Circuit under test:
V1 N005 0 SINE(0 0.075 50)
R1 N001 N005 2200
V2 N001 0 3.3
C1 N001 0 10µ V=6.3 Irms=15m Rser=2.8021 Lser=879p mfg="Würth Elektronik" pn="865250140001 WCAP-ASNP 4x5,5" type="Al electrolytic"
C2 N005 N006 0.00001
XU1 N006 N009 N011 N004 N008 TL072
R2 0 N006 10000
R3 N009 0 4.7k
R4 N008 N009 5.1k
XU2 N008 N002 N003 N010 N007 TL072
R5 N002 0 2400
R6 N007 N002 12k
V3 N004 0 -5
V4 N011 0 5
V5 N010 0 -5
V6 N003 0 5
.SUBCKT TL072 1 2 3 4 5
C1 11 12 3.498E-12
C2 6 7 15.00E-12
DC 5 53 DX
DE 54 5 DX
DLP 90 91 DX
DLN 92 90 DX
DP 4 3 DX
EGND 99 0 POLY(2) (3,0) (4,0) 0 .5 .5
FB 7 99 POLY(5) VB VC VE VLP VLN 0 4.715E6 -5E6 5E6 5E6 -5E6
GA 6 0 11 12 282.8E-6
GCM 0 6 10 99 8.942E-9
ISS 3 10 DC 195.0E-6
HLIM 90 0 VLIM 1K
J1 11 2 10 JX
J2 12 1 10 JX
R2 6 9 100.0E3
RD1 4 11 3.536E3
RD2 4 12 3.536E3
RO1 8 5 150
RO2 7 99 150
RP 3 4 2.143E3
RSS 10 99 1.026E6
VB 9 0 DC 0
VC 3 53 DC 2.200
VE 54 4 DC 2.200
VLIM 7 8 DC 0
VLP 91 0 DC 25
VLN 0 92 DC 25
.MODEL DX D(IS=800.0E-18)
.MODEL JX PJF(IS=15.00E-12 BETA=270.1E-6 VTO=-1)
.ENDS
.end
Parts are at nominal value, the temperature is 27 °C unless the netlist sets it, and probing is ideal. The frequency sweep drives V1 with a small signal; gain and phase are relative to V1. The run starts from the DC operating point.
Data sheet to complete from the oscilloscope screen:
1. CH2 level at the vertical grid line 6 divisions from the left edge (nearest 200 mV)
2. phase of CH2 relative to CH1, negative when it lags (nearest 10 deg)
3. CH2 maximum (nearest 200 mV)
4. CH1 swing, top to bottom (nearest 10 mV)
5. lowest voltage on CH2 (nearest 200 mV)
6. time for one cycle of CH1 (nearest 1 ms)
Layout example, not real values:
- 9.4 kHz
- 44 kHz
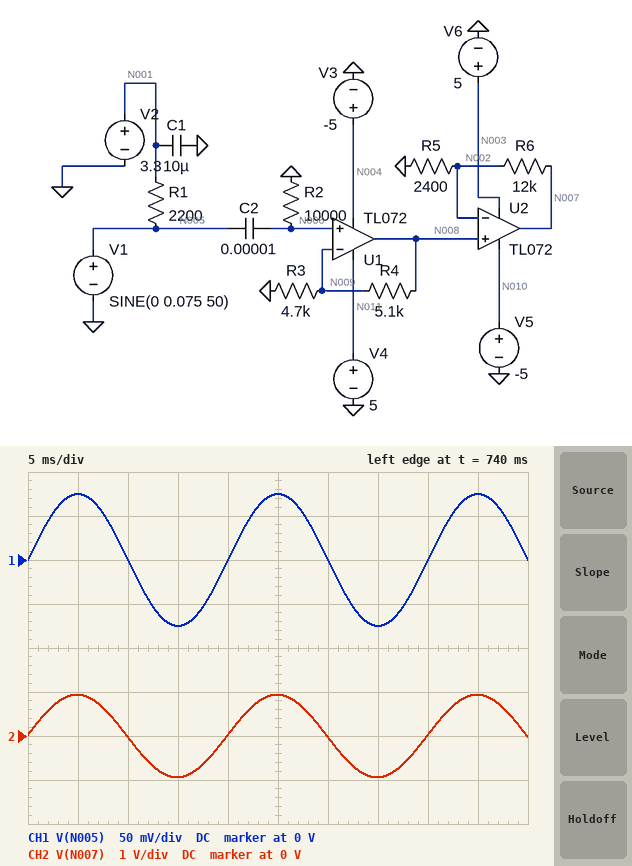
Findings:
- 0 V
- 0 deg
- 1.0 V
- 150 mV
- -1.0 V
- 20 ms
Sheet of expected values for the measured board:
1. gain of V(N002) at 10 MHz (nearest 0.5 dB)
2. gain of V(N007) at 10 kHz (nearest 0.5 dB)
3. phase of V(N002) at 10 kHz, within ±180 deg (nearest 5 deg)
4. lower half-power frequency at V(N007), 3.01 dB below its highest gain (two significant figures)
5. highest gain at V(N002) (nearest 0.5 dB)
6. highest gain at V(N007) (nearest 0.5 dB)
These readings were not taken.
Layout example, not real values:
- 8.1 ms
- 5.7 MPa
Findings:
- -44.0 dB
- 22.0 dB
- 0 deg
- 1.6 Hz
- 6.5 dB
- 22.0 dB
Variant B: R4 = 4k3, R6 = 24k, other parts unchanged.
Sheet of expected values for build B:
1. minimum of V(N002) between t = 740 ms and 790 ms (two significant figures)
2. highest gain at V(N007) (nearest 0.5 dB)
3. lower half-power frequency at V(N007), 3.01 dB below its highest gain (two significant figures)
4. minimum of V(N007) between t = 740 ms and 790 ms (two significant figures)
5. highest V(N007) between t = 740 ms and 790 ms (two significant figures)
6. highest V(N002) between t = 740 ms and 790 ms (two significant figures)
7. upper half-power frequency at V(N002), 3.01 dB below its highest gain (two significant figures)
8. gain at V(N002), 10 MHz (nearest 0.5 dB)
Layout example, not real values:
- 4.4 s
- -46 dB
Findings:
- -140 mV
- 26.5 dB
- 1.6 Hz
- -1.6 V
- 1.6 V
- 140 mV
- 320 kHz
- -49.5 dB
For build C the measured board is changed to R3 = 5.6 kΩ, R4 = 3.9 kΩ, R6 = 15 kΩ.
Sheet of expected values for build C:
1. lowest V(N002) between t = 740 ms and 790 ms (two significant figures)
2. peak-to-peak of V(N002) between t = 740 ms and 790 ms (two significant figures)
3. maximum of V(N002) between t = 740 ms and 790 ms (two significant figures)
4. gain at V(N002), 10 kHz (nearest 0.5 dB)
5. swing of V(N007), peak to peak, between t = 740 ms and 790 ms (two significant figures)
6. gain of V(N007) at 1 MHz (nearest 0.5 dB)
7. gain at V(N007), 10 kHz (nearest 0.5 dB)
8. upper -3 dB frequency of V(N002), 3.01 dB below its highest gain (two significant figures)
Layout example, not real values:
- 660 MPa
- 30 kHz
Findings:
- -130 mV
- 250 mV
- 130 mV
- 4.5 dB
- 1.8 V
- 14.5 dB
- 22.0 dB
- 500 kHz
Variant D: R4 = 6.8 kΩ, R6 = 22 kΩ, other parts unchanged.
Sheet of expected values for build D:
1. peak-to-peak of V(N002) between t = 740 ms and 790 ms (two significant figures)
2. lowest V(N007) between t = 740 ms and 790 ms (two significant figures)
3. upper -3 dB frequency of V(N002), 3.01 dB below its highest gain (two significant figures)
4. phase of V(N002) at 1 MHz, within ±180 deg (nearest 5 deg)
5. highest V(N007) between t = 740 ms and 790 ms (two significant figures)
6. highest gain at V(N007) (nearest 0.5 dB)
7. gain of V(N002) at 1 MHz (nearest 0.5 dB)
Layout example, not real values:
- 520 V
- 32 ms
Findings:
- 370 mV
- -1.9 V
- 340 kHz
- -120 deg
- 1.9 V
- 28.0 dB
- -3.0 dB
